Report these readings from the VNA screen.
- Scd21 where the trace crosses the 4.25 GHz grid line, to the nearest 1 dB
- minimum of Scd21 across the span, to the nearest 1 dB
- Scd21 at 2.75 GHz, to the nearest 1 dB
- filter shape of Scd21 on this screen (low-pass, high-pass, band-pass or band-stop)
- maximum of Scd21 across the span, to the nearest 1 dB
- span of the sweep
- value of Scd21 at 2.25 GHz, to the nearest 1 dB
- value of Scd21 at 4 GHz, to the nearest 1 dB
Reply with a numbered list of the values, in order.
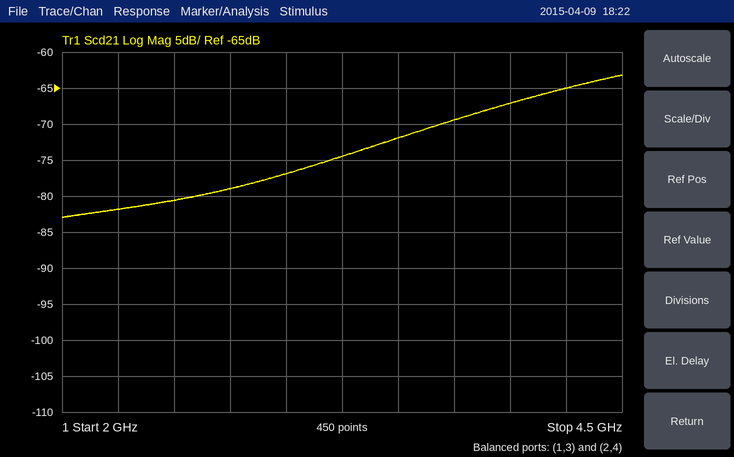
1. -65 dB
2. -83 dB
3. -79 dB
4. high-pass
5. -63 dB
6. 2.5 GHz
7. -82 dB
8. -67 dB
